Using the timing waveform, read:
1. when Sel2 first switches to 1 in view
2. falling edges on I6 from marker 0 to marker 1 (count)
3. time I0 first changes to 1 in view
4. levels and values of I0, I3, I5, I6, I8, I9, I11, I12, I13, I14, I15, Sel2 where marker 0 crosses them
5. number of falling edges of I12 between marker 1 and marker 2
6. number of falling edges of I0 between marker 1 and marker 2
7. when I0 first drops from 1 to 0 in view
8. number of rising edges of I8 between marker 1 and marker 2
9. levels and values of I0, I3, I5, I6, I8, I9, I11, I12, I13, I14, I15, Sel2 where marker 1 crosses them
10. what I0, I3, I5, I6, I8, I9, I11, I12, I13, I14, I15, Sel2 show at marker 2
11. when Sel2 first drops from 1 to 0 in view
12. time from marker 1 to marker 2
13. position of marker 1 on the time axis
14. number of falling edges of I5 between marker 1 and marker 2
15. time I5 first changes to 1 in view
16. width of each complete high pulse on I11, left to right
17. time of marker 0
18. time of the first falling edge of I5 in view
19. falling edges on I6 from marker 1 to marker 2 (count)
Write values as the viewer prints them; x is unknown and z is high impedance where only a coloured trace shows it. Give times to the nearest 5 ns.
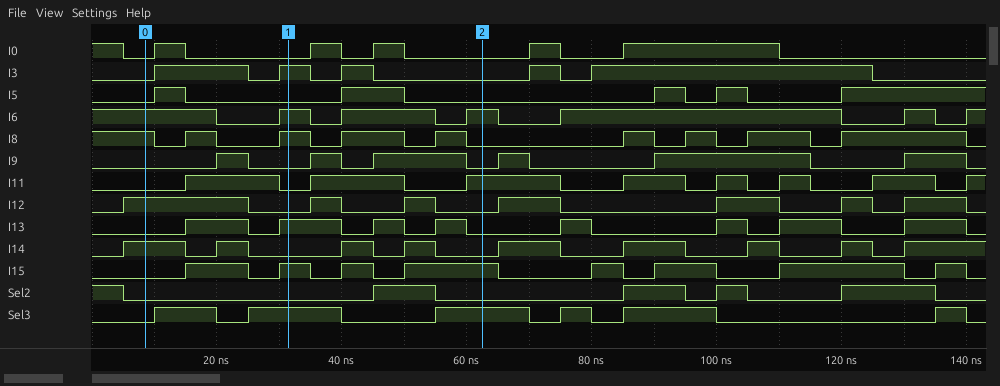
45 ns
1
10 ns
I0=0, I3=0, I5=0, I6=1, I8=1, I9=0, I11=0, I12=1, I13=0, I14=1, I15=0, Sel2=0
2
2
5 ns
2
I0=0, I3=1, I5=0, I6=1, I8=1, I9=0, I11=0, I12=0, I13=1, I14=0, I15=1, Sel2=0
I0=0, I3=0, I5=0, I6=1, I8=0, I9=0, I11=1, I12=0, I13=0, I14=0, I15=1, Sel2=0
5 ns
30 ns
30 ns
1
10 ns
15 ns, 15 ns, 15 ns, 10 ns, 5 ns, 5 ns, 10 ns
10 ns
15 ns
2
